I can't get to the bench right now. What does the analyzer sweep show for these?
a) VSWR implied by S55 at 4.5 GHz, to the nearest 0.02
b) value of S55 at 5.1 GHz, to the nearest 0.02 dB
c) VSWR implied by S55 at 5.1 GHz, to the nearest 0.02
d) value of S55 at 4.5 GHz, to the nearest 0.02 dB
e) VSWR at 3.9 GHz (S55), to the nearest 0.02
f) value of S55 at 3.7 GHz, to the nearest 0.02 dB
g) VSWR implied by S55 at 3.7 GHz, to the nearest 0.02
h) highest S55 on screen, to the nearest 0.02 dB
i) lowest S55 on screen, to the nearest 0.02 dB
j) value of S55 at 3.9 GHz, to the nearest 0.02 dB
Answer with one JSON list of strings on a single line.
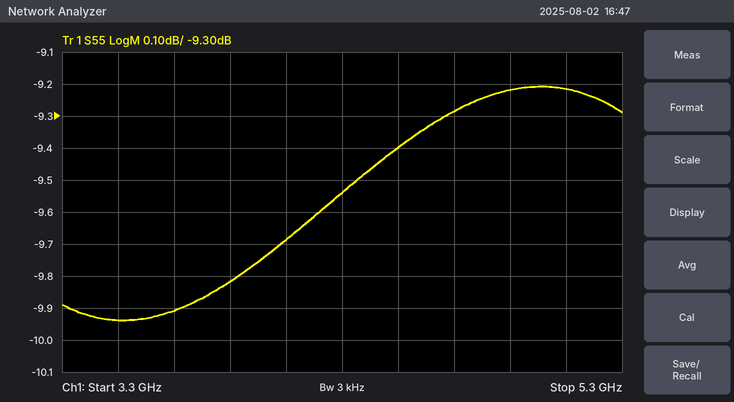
["2.02", "-9.22 dB", "2.06", "-9.40 dB", "1.96", "-9.90 dB", "1.94", "-9.20 dB", "-9.94 dB", "-9.82 dB"]
